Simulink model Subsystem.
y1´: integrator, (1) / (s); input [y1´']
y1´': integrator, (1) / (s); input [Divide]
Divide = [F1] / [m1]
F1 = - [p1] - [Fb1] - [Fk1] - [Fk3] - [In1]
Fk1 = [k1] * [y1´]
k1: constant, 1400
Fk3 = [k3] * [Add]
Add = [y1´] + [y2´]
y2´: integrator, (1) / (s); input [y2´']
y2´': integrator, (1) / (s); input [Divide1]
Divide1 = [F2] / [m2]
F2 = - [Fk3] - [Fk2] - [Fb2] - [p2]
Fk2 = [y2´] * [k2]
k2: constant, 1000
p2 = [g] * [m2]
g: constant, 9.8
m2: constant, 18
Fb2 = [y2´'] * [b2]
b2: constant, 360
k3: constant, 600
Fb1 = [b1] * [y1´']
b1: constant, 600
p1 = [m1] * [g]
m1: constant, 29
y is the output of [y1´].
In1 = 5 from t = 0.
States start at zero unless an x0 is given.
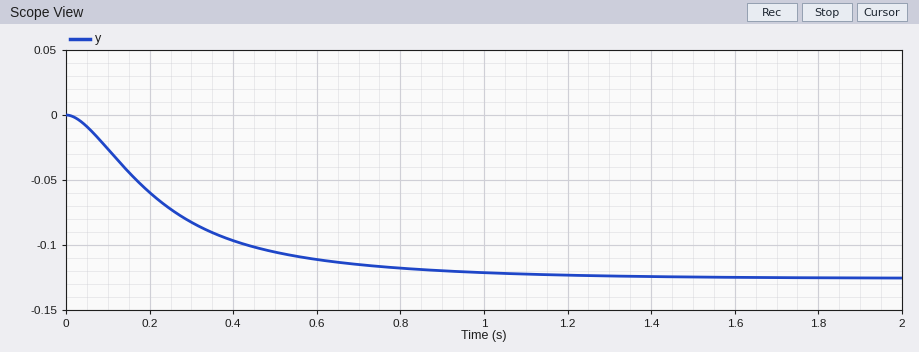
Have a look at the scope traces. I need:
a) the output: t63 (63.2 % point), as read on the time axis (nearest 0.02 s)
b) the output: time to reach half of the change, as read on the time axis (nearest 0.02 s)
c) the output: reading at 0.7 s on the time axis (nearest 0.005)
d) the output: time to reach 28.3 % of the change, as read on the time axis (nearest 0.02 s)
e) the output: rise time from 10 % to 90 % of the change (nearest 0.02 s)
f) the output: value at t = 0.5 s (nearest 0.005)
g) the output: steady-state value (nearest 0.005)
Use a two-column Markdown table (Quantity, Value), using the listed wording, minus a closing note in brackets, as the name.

| Quantity | Value |
|---|---|
| the output: t63 (63.2 % point), as read on the time axis | 0.28 s |
| the output: time to reach half of the change, as read on the time axis | 0.22 s |
| the output: reading at 0.7 s on the time axis | -0.115 |
| the output: time to reach 28.3 % of the change, as read on the time axis | 0.12 s |
| the output: rise time from 10 % to 90 % of the change | 0.58 s |
| the output: value at t = 0.5 s | -0.105 |
| the output: steady-state value | -0.125 |
